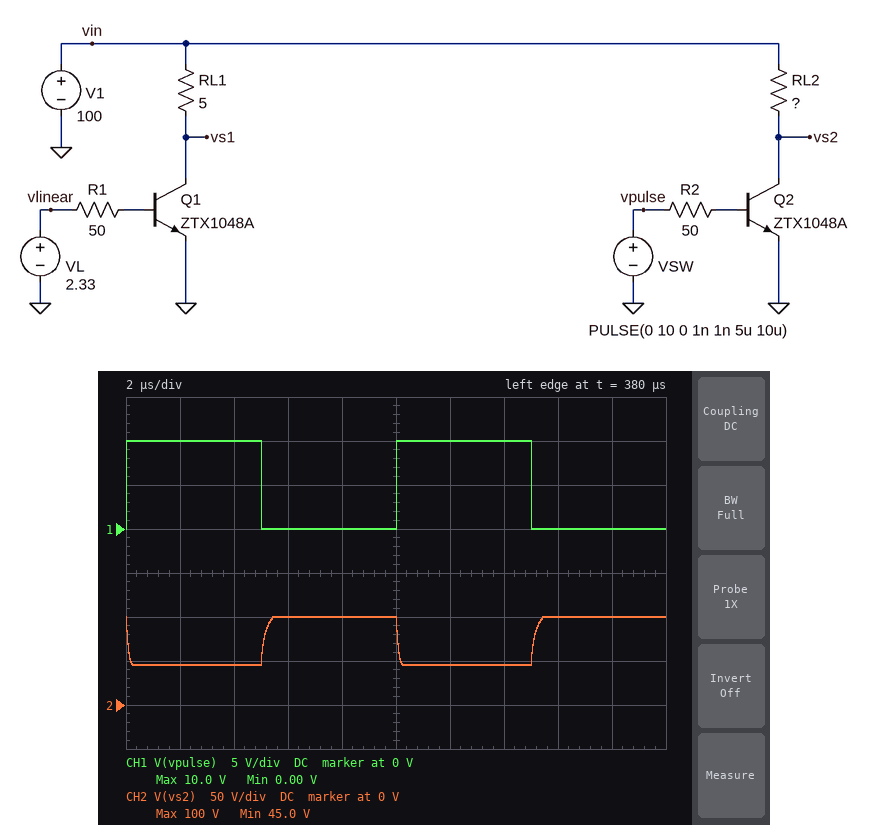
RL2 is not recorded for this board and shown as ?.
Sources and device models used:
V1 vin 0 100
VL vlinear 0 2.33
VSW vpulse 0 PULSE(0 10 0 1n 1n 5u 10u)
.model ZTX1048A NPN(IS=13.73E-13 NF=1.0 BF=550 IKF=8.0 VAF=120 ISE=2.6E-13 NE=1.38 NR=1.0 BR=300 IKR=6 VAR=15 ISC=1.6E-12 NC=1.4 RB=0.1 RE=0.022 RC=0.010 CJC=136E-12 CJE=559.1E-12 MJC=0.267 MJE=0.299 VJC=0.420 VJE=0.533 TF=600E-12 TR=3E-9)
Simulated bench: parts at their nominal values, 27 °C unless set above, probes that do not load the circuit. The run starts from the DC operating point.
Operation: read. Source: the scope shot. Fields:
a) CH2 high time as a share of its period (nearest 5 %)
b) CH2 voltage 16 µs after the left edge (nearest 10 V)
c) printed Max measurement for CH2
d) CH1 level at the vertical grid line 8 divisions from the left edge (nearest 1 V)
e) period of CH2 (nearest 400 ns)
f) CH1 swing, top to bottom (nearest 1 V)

50 %
100 V
100 V
0 V
10.0 µs
10 V
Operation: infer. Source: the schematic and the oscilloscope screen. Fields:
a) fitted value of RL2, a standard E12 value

1.8 Ω
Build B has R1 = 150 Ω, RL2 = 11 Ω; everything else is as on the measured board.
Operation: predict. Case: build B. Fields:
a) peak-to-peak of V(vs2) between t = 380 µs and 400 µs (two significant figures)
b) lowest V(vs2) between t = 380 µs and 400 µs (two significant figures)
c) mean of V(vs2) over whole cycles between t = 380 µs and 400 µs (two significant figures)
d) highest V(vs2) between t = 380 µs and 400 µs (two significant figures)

100 V
320 mV
43 V
100 V
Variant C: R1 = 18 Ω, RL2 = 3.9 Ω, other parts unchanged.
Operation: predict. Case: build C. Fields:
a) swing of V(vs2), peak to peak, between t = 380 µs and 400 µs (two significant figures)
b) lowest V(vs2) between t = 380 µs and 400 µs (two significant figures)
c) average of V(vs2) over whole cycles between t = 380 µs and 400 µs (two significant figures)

92 V
8.0 V
53 V
